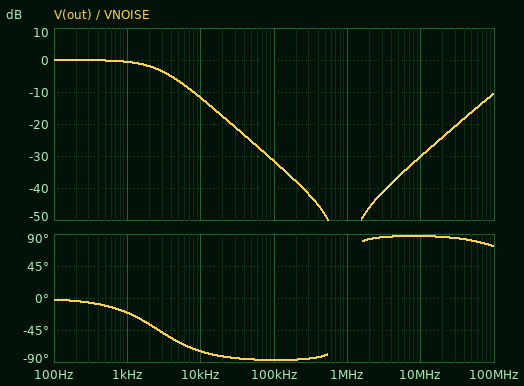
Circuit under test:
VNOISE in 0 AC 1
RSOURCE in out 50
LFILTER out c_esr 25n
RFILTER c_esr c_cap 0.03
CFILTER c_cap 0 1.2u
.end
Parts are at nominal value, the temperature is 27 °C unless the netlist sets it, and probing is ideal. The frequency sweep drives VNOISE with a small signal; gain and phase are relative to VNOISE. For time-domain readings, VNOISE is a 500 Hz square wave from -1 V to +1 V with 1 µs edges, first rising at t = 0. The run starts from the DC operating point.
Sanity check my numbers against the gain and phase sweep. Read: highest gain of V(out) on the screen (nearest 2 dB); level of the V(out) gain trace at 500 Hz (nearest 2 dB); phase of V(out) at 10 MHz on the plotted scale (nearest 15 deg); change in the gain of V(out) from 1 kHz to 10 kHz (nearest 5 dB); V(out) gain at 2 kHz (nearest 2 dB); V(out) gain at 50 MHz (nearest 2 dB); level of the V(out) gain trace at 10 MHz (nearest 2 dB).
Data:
0 dB
0 dB
90 deg
-10 dB
-2 dB
-16 dB
-30 dB
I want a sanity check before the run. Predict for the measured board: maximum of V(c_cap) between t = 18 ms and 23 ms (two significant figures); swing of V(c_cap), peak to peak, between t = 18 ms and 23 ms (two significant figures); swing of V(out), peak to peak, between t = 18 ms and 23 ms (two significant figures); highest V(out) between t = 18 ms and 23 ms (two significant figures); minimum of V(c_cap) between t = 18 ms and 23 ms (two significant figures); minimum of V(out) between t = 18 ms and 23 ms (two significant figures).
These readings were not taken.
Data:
1.0 V
2.0 V
2.0 V
1.0 V
-1.0 V
-1.0 V
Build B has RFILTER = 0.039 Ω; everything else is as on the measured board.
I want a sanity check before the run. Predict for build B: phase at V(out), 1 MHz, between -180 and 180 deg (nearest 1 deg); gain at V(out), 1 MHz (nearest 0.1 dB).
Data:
32 deg
-60.7 dB
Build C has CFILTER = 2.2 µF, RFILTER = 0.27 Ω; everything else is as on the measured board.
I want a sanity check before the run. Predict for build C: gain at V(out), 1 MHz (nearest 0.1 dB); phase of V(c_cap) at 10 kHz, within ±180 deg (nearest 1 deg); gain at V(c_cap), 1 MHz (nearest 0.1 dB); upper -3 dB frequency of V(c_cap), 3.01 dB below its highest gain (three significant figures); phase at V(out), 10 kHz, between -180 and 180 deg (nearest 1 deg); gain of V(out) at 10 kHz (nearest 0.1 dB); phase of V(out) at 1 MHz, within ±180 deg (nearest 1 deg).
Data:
-45.0 dB
-82 deg
-56.8 dB
1.44 kHz
-80 deg
-16.9 dB
17 deg
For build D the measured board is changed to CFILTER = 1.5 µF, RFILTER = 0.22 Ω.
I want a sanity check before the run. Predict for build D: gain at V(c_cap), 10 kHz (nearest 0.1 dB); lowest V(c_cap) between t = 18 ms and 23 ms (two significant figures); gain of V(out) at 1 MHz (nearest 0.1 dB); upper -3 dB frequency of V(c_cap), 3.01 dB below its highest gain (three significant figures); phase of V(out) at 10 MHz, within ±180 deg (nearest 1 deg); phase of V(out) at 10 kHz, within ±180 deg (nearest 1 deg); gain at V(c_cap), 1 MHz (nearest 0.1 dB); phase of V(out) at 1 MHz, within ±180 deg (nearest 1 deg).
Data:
-13.7 dB
-1.0 V
-46.9 dB
2.11 kHz
80 deg
-77 deg
-53.5 dB
13 deg
